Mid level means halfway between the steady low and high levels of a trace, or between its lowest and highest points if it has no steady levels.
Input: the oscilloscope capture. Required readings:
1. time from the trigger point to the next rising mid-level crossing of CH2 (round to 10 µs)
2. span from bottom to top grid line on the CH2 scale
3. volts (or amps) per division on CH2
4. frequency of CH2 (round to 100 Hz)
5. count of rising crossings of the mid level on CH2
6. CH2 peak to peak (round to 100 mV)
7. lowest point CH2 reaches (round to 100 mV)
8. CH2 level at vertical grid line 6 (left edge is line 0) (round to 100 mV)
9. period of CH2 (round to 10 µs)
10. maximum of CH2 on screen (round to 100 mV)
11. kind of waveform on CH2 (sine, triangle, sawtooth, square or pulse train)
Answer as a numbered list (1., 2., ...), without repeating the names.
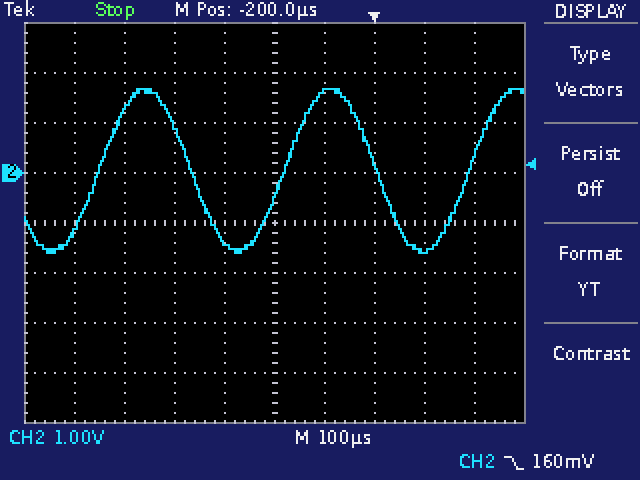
1. 190 µs
2. 8 V
3. 1 V
4. 2.7 kHz
5. 3
6. 3.3 V
7. -1.6 V
8. 1.6 V
9. 370 µs
10. 1.7 V
11. sine
